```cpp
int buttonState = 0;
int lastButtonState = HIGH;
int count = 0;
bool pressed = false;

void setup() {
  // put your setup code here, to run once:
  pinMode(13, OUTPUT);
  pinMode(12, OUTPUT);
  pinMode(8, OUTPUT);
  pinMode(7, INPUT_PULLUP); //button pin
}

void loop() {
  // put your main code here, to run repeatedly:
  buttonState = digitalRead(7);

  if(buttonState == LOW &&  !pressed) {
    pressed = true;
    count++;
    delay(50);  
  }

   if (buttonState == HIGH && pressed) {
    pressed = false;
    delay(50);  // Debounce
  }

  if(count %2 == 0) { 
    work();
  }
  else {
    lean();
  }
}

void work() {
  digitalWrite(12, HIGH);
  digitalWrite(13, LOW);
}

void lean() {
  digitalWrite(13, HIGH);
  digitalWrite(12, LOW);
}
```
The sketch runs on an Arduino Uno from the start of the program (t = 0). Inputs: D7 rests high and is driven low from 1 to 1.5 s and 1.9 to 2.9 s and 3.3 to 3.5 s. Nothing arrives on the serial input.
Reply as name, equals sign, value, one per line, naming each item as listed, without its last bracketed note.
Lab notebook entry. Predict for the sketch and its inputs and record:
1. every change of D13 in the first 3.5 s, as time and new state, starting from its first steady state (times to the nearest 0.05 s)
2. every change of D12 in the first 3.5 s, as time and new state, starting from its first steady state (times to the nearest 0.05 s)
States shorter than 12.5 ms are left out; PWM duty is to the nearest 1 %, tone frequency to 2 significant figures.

every change of D13 in the first 3.5 s, as time and new state, starting from its first steady state = 0 s low; 1.05 s high; 1.95 s low; 3.35 s high
every change of D12 in the first 3.5 s, as time and new state, starting from its first steady state = 0 s high; 1.05 s low; 1.95 s high; 3.35 s low
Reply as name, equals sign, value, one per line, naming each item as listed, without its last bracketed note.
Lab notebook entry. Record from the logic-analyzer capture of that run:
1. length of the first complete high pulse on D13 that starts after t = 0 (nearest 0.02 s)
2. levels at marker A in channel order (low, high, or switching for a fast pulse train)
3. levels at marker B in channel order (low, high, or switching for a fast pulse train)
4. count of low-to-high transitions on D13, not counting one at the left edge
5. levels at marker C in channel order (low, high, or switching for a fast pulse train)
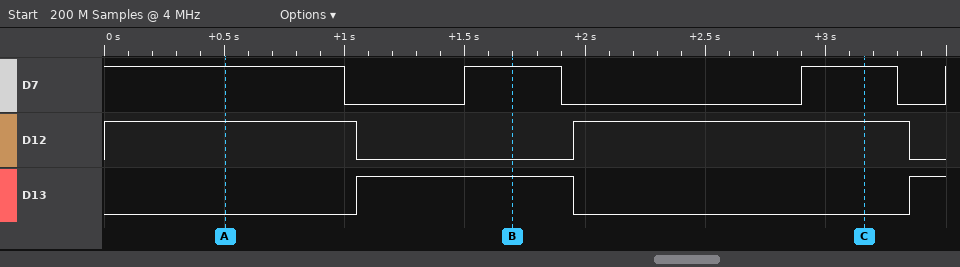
length of the first complete high pulse on D13 that starts after t = 0 = 0.90 s
levels at marker A in channel order = D7 high, D12 high, D13 low
levels at marker B in channel order = D7 high, D12 low, D13 high
count of low-to-high transitions on D13, not counting one at the left edge = 2
levels at marker C in channel order = D7 high, D12 high, D13 low
